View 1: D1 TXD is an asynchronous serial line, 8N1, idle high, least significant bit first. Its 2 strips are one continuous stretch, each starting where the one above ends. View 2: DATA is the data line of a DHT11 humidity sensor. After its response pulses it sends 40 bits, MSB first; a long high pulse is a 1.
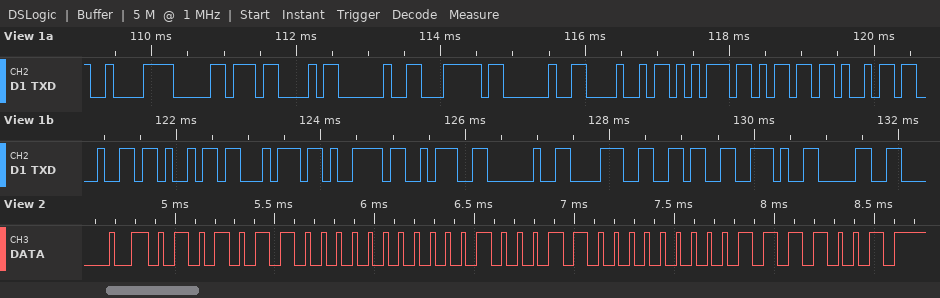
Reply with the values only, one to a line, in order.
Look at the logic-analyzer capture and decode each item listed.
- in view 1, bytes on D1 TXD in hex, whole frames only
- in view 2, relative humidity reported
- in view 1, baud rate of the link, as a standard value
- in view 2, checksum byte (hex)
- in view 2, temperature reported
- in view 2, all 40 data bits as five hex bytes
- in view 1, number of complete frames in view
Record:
0xC2 0xB0 0x43 0x20 0x7C 0x20 0x48 0x75 0x6D 0x69 0x64 0x69 0x74 0x79 0x3A 0x20 0x38 0x36 0x2E 0x30
86 %
9600 baud
0x79
35.0 °C
56 00 23 00 79
20
